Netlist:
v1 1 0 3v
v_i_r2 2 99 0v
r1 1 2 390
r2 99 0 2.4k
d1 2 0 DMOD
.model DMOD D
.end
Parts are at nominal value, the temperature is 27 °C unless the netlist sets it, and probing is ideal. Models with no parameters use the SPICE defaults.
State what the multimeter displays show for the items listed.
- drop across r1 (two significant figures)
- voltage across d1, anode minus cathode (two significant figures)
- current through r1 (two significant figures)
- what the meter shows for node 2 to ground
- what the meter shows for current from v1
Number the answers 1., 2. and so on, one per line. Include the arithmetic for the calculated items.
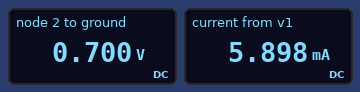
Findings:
1. 3 V - 700 mV = 2.3 V
2. 700 mV = 700 mV
3. (3 V - 700 mV) / 390 Ω = 5.9 mA
4. 0.700 V
5. 5.898 mA
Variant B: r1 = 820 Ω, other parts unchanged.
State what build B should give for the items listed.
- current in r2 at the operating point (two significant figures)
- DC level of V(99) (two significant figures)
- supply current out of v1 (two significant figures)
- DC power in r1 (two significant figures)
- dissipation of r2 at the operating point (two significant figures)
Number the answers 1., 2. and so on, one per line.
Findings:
1. 280 µA
2. 680 mV
3. 2.8 mA
4. 6.6 mW
5. 190 µW
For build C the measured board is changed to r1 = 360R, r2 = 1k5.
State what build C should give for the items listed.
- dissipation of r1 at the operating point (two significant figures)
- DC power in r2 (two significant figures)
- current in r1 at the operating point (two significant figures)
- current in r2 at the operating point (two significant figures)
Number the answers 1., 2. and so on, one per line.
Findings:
1. 15 mW
2. 330 µW
3. 6.4 mA
4. 470 µA
